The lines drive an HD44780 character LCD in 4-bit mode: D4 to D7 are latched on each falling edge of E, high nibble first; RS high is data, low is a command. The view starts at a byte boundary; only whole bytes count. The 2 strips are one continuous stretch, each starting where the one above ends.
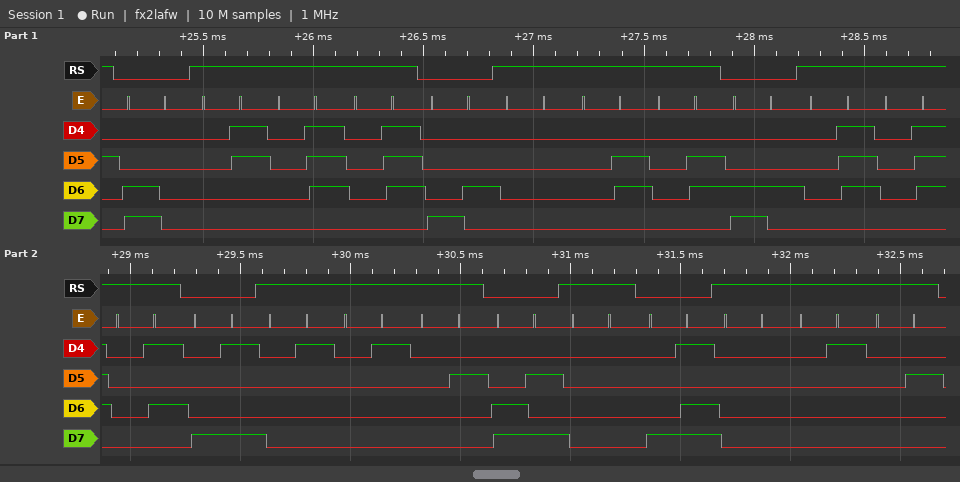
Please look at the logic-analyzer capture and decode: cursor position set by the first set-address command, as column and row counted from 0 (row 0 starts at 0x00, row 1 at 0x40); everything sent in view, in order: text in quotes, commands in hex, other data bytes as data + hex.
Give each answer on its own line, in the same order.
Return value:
column 0, row 1
0xC0 data 03 07 07 0x84 data 00 06 06 0xC4 data 07 07 05 0x89 data 01 01 02 0xCA data 00 0x8D data 00 01 02
